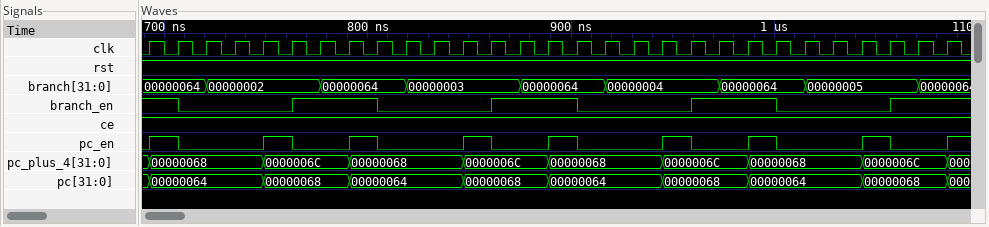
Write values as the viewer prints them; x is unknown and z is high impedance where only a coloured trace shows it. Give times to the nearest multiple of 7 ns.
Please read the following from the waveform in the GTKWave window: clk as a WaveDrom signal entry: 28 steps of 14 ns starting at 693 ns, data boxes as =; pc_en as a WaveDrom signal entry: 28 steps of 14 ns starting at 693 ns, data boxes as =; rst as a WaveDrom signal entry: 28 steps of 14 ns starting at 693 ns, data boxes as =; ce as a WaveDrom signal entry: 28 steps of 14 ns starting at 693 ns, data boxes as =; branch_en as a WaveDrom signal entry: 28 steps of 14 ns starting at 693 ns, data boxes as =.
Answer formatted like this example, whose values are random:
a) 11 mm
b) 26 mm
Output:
a) {name: 'clk', wave: 'p...........................'}
b) {name: 'pc_en', wave: '10..10.10..10.10..10.10..10.'}
c) {name: 'rst', wave: '1...........................'}
d) {name: 'ce', wave: '1...........................'}
e) {name: 'branch_en', wave: '10...1..0...1..0...1..0...1.'}
